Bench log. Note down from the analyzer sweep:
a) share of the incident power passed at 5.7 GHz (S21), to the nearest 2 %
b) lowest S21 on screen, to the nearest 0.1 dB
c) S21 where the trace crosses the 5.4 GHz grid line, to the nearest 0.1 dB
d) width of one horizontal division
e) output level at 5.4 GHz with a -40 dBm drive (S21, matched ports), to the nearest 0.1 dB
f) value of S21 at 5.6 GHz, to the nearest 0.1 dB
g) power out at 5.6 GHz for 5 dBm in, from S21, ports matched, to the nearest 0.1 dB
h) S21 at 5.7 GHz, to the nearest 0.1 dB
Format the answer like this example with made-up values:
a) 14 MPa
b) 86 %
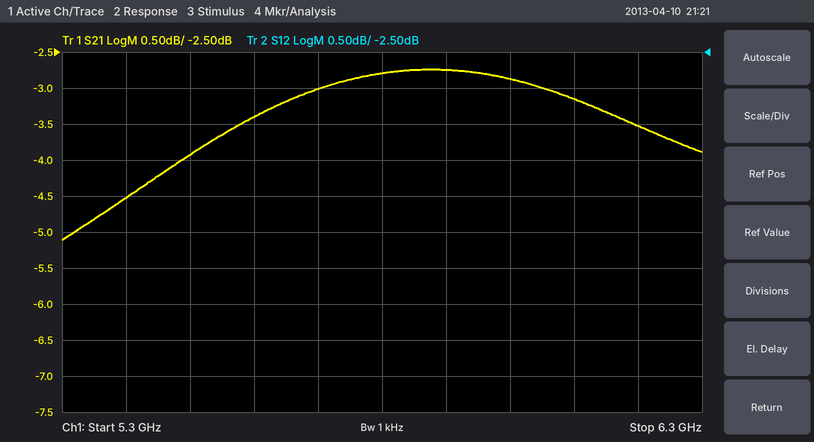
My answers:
a) 50 %
b) -5.1 dB
c) -4.5 dB
d) 100 MHz
e) -44.5 dBm
f) -3.4 dB
g) 1.6 dBm
h) -3.0 dB
